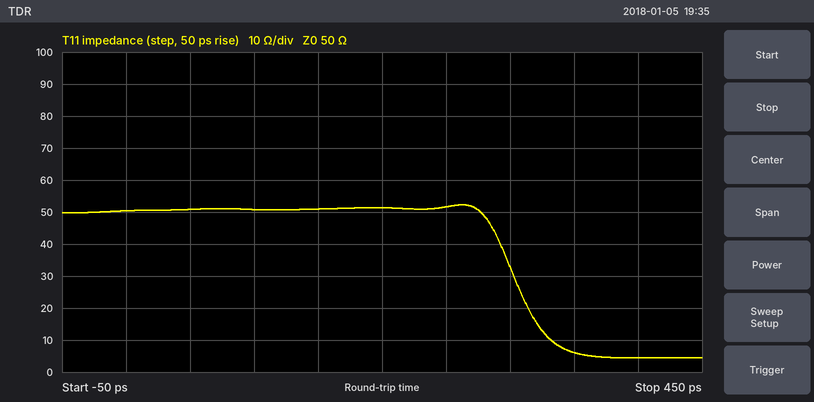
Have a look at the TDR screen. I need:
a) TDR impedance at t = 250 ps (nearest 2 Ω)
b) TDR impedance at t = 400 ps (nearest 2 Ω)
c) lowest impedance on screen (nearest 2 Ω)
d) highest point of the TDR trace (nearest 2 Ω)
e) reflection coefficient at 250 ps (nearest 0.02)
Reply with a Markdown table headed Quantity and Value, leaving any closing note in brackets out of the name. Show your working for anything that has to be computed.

| Quantity | Value |
|---|---|
| TDR impedance at t = 250 ps | 52 Ω |
| TDR impedance at t = 400 ps | 4 Ω |
| lowest impedance on screen | 4 Ω |
| highest point of the TDR trace | 52 Ω |
| reflection coefficient at 250 ps | (52 − 50)/(52 + 50) ≈ +0.02 |
